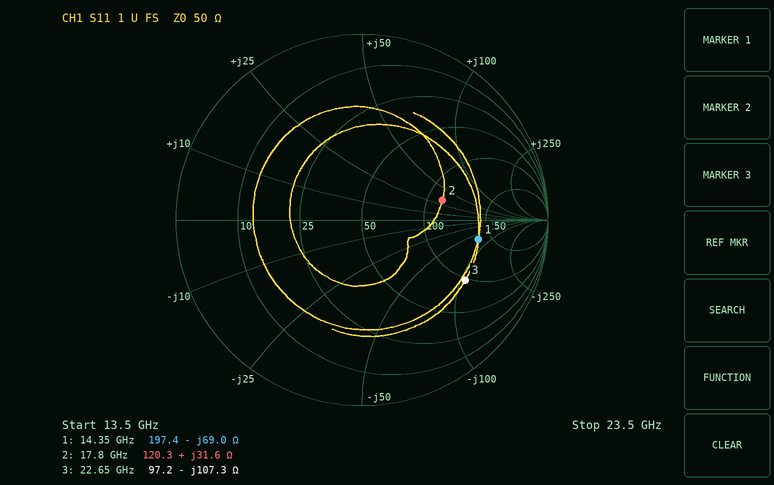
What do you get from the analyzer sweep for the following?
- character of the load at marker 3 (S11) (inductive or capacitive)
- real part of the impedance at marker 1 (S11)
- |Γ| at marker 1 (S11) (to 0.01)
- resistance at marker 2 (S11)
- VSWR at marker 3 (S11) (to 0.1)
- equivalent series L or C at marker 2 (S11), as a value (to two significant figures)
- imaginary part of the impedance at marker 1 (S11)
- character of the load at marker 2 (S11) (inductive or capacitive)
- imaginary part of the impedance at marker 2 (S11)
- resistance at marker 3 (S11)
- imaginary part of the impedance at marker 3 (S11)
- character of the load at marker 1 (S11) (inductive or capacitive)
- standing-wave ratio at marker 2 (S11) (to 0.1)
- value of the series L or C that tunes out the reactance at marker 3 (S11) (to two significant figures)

capacitive
197.4 Ω
0.63
120.3 Ω
4.6
280 pH
-69.0 Ω
inductive
+31.6 Ω
97.2 Ω
-107.3 Ω
capacitive
2.6
750 pH
